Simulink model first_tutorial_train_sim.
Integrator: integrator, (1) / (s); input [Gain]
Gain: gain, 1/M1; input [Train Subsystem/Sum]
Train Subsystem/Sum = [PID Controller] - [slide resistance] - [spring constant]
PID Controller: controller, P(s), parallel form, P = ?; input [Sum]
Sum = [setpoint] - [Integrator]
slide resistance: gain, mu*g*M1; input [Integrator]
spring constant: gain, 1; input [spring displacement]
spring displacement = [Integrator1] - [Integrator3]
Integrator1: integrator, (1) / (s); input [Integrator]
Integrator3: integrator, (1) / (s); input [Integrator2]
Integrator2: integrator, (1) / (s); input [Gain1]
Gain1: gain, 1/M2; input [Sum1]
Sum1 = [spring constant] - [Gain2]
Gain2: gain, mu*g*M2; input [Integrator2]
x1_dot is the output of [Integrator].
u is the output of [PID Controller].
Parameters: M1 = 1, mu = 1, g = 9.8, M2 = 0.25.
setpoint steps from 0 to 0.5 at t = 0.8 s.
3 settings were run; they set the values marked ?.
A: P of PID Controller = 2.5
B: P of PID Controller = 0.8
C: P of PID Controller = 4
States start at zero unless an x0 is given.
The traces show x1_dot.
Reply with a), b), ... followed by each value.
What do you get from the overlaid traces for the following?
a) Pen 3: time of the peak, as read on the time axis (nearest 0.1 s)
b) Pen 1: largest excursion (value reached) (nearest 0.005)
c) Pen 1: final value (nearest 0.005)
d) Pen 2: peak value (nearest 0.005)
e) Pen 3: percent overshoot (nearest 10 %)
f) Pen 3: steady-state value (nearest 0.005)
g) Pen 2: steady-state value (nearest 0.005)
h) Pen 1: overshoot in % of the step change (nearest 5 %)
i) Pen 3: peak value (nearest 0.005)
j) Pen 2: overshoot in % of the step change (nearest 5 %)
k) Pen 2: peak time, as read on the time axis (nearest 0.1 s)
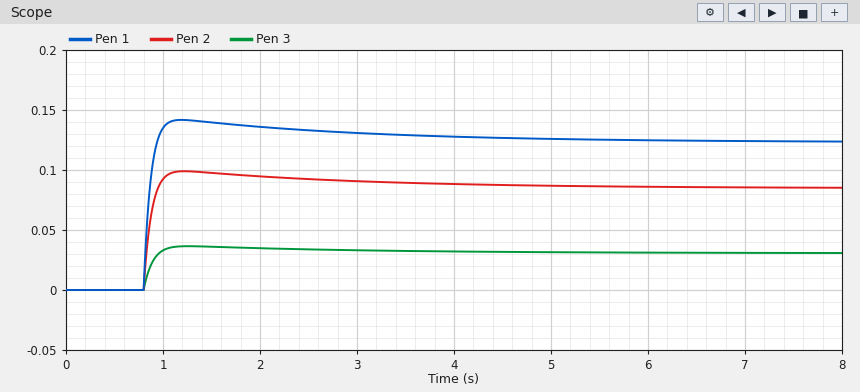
a) 1.3 s
b) 0.140
c) 0.125
d) 0.100
e) 20 %
f) 0.030
g) 0.085
h) 15 %
i) 0.035
j) 15 %
k) 1.2 s
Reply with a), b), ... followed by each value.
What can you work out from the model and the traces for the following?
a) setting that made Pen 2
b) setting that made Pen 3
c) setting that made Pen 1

a) A
b) B
c) C
